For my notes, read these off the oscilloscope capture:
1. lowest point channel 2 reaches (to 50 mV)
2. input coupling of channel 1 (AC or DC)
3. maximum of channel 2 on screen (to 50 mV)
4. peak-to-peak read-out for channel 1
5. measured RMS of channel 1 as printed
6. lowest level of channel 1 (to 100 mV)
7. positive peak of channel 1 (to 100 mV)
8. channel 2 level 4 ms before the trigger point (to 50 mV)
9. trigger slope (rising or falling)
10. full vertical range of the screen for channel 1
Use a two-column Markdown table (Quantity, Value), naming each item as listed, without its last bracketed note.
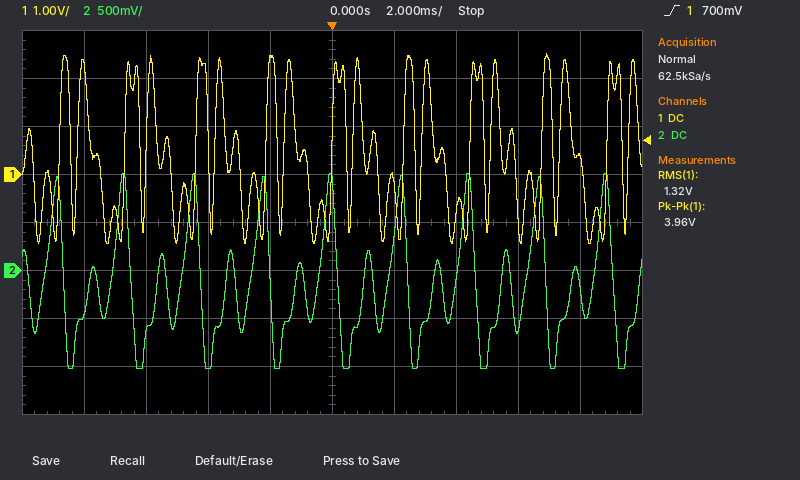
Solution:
| Quantity | Value |
|---|---|
| lowest point channel 2 reaches | -1.00 V |
| input coupling of channel 1 | DC |
| maximum of channel 2 on screen | 1.00 V |
| peak-to-peak read-out for channel 1 | 3.96 V |
| measured RMS of channel 1 as printed | 1.32 V |
| lowest level of channel 1 | -1.4 V |
| positive peak of channel 1 | 2.5 V |
| channel 2 level 4 ms before the trigger point | -1.00 V |
| trigger slope | rising |
| full vertical range of the screen for channel 1 | 8 V |
